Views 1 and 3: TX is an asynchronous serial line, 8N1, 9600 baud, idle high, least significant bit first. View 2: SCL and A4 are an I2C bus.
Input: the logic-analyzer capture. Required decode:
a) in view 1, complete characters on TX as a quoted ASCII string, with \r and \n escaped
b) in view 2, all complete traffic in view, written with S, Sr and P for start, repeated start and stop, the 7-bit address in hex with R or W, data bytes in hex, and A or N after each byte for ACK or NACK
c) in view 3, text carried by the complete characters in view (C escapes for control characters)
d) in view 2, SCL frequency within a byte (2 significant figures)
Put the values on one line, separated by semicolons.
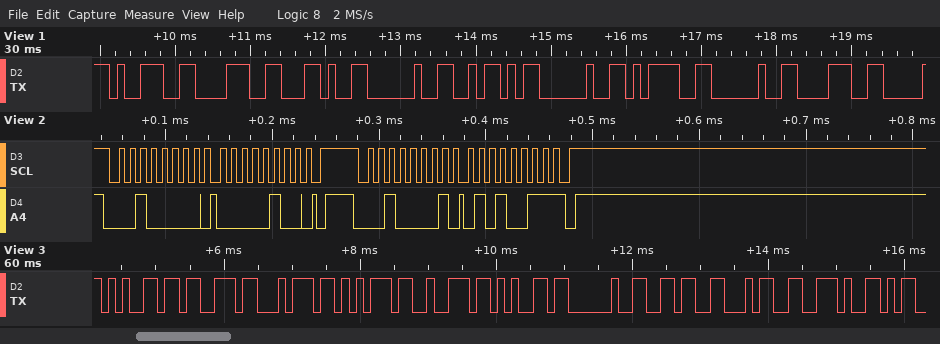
"98, Z = 8"; S 10W A 04 A P S 10R A 53 N P; "esture 64."; 100 kHz
